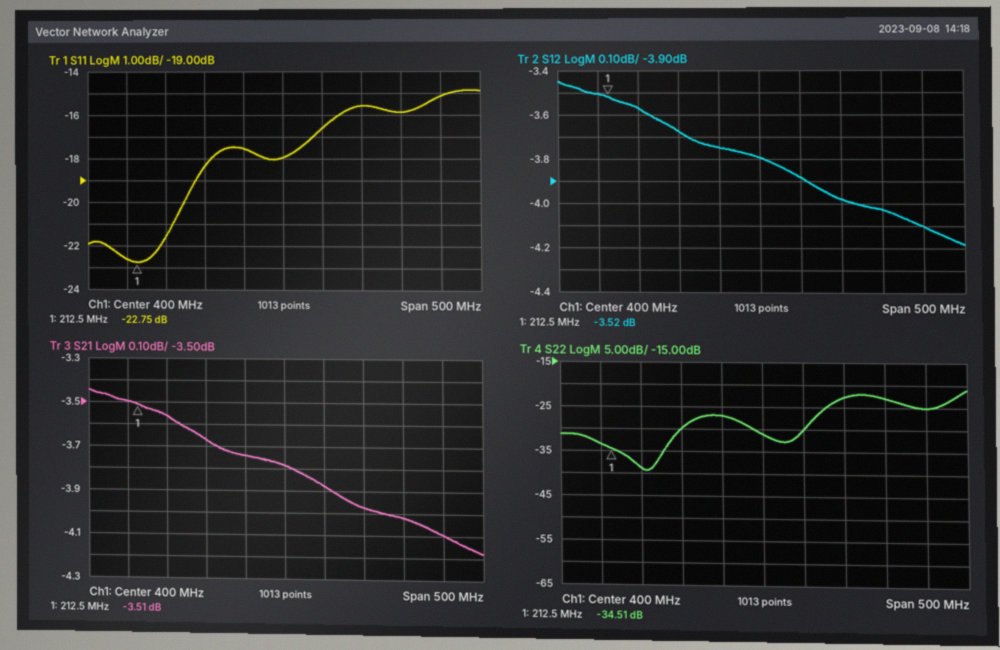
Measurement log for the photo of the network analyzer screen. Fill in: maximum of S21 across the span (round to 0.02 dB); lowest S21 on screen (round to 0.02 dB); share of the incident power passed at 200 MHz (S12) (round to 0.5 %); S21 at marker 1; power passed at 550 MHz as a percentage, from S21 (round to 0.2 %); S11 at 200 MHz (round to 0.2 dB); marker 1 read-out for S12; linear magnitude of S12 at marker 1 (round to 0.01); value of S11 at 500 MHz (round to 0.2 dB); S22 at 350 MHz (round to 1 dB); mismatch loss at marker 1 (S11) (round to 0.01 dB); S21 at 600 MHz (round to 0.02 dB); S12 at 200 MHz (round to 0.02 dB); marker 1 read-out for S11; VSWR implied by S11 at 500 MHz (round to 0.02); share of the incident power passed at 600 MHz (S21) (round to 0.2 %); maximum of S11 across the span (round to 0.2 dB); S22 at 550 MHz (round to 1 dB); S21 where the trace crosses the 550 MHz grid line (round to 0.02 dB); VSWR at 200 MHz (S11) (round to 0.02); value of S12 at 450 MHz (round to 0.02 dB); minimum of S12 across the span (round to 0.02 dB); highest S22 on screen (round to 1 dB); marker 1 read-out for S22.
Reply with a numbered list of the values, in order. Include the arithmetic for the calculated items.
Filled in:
1. -3.44 dB
2. -4.18 dB
3. 10^(-3.5/10) ≈ 44.7 %, so 44.5 % to the nearest 0.5 %
4. -3.51 dB
5. 10^(-4.02/10) ≈ 39.6 %
6. -22.6 dB
7. -3.52 dB
8. 10^(-3.52/20) ≈ 0.67
9. -15.6 dB
10. -27 dB
11. −10 log10(1 − 10^(-22.75/10)) ≈ 0.02 dB
12. -4.10 dB
13. -3.50 dB
14. -22.75 dB
15. |Γ| = 10^(-15.6/20) = 0.1660; VSWR = (1 + 0.1660)/(1 − 0.1660) ≈ 1.40
16. 10^(-4.1/10) ≈ 38.9 %, so 39.0 % to the nearest 0.2 %
17. -14.8 dB
18. -23 dB
19. -4.02 dB
20. |Γ| = 10^(-22.6/20) = 0.0741; VSWR = (1 + 0.0741)/(1 − 0.0741) ≈ 1.16
21. -3.88 dB
22. -4.18 dB
23. -21 dB
24. -34.51 dB
